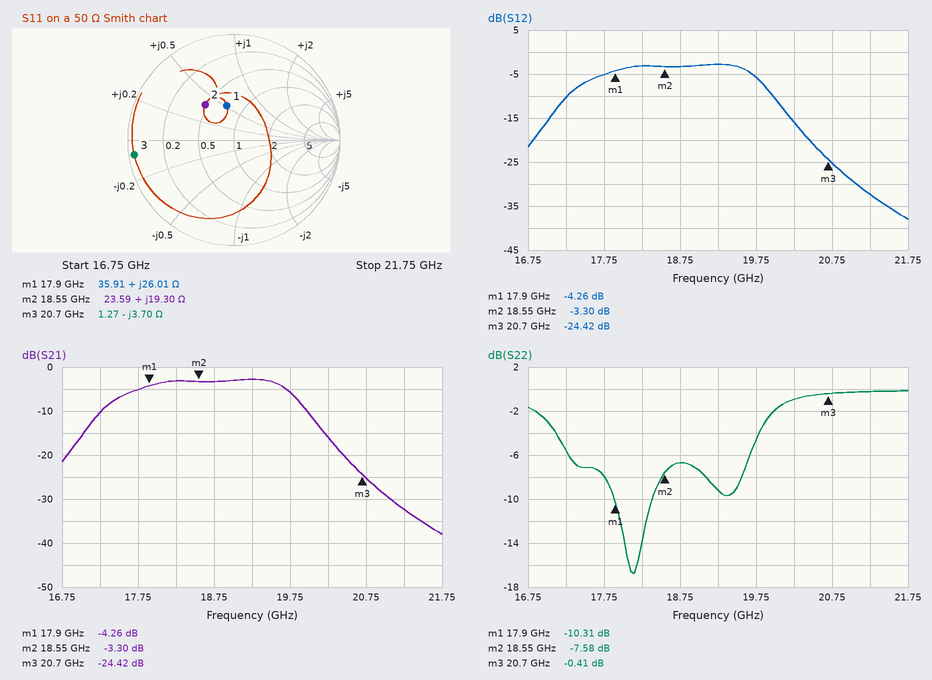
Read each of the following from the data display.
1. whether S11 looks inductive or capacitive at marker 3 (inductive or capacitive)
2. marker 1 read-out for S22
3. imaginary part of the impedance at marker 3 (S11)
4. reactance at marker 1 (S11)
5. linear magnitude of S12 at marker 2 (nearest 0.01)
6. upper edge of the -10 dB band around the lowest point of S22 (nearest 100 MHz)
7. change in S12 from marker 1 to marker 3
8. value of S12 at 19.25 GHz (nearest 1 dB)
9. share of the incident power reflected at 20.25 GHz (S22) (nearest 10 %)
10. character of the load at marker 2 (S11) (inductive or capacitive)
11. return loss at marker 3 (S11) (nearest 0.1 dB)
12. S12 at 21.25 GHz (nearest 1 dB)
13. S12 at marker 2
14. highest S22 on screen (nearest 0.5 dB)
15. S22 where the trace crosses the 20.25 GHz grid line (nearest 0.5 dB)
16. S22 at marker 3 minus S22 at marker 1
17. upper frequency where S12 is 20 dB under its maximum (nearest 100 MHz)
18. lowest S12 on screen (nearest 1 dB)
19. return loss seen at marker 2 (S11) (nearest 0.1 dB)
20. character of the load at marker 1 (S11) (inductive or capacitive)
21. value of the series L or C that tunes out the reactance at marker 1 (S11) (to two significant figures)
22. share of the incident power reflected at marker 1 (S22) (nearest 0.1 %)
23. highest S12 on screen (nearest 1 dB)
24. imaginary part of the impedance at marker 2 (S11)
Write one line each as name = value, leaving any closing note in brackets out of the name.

whether S11 looks inductive or capacitive at marker 3 = capacitive
marker 1 read-out for S22 = -10.31 dB
imaginary part of the impedance at marker 3 = -3.70 Ω
reactance at marker 1 = +26.01 Ω
linear magnitude of S12 at marker 2 = 0.68
upper edge of the -10 dB band around the lowest point of S22 = 18.4 GHz
change in S12 from marker 1 to marker 3 = -20.16 dB
value of S12 at 19.25 GHz = -3 dB
share of the incident power reflected at 20.25 GHz (S22) = 80 %
character of the load at marker 2 (S11) = inductive
return loss at marker 3 (S11) = 0.4 dB
S12 at 21.25 GHz = -32 dB
S12 at marker 2 = -3.30 dB
highest S22 on screen = 0.0 dB
S22 where the trace crosses the 20.25 GHz grid line = -1.0 dB
S22 at marker 3 minus S22 at marker 1 = 9.90 dB
upper frequency where S12 is 20 dB under its maximum = 20.6 GHz
lowest S12 on screen = -38 dB
return loss seen at marker 2 (S11) = 7.3 dB
character of the load at marker 1 (S11) = inductive
value of the series L or C that tunes out the reactance at marker 1 (S11) = 340 fF
share of the incident power reflected at marker 1 (S22) = 9.3 %
highest S12 on screen = -3 dB
imaginary part of the impedance at marker 2 = +19.30 Ω
